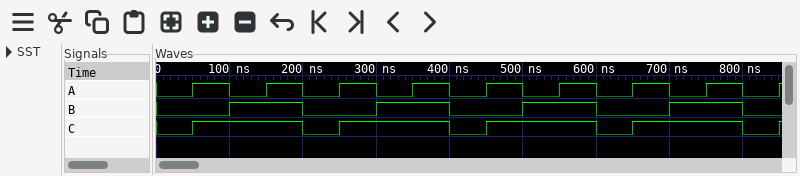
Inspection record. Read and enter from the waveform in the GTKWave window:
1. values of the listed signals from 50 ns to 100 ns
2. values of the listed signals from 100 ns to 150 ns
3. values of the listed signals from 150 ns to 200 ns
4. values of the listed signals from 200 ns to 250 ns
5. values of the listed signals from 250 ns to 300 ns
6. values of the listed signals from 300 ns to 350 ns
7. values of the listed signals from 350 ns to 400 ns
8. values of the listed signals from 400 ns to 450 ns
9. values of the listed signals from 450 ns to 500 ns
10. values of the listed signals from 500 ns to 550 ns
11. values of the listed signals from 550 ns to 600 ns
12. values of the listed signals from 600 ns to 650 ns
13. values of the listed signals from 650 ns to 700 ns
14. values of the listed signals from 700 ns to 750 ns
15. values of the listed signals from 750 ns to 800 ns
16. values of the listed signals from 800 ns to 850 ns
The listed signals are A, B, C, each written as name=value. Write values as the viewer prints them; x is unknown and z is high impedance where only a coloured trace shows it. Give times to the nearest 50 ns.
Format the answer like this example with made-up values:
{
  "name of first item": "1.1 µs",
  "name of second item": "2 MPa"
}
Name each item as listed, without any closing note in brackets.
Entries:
{
  "values of the listed signals from 50 ns to 100 ns": "A=1, B=0, C=1",
  "values of the listed signals from 100 ns to 150 ns": "A=0, B=1, C=1",
  "values of the listed signals from 150 ns to 200 ns": "A=1, B=1, C=1",
  "values of the listed signals from 200 ns to 250 ns": "A=0, B=0, C=0",
  "values of the listed signals from 250 ns to 300 ns": "A=1, B=0, C=1",
  "values of the listed signals from 300 ns to 350 ns": "A=0, B=1, C=1",
  "values of the listed signals from 350 ns to 400 ns": "A=1, B=1, C=1",
  "values of the listed signals from 400 ns to 450 ns": "A=0, B=0, C=0",
  "values of the listed signals from 450 ns to 500 ns": "A=1, B=0, C=1",
  "values of the listed signals from 500 ns to 550 ns": "A=0, B=1, C=1",
  "values of the listed signals from 550 ns to 600 ns": "A=1, B=1, C=1",
  "values of the listed signals from 600 ns to 650 ns": "A=0, B=0, C=0",
  "values of the listed signals from 650 ns to 700 ns": "A=1, B=0, C=1",
  "values of the listed signals from 700 ns to 750 ns": "A=0, B=1, C=1",
  "values of the listed signals from 750 ns to 800 ns": "A=1, B=1, C=1",
  "values of the listed signals from 800 ns to 850 ns": "A=0, B=0, C=0"
}
